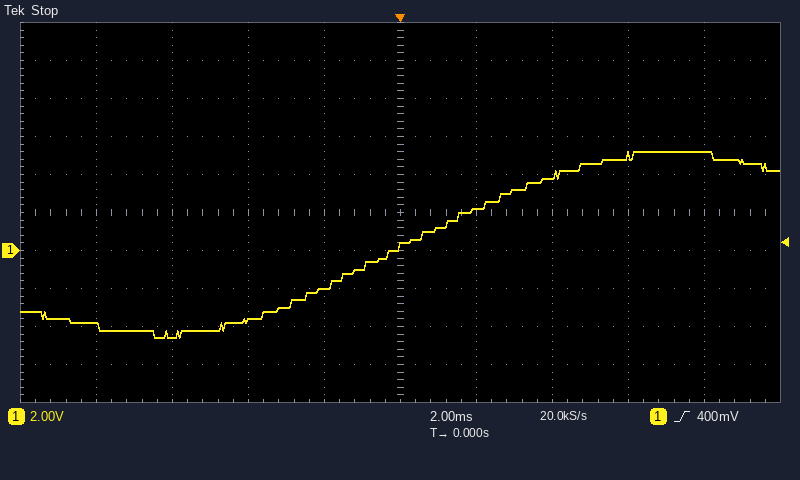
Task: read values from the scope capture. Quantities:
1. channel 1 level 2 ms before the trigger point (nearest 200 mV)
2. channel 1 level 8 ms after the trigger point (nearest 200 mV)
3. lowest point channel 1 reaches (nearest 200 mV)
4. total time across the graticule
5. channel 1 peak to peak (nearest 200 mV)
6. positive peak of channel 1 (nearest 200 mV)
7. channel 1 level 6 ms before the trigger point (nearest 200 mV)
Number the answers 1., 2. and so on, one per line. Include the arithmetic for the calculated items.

1. -2.0 V
2. 5.2 V
3. -4.6 V
4. 20 ms
5. 5.2 V − (-4.6 V) = 9.8 V
6. 5.2 V
7. -4.6 V
